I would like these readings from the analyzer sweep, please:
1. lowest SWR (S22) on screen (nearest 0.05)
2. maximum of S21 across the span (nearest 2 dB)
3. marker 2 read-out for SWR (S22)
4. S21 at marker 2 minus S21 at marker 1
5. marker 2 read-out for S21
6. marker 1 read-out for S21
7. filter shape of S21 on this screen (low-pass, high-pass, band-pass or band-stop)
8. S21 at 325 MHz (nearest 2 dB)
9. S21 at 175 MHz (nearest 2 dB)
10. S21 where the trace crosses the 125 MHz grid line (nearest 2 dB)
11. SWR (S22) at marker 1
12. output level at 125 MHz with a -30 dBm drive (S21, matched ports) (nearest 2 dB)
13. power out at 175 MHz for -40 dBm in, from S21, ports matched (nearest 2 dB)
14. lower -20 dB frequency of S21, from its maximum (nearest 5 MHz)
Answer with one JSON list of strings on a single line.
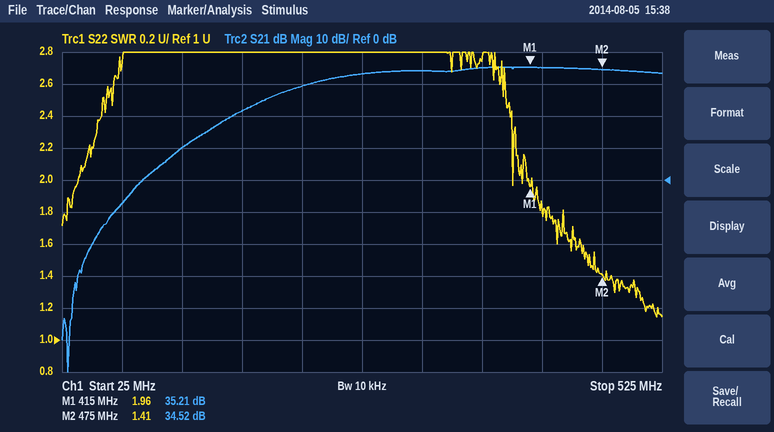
["1.15", "36 dB", "1.41", "-0.69 dB", "34.52 dB", "35.21 dB", "high-pass", "34 dB", "22 dB", "10 dB", "1.96", "-20 dBm", "-18 dBm", "145 MHz"]
